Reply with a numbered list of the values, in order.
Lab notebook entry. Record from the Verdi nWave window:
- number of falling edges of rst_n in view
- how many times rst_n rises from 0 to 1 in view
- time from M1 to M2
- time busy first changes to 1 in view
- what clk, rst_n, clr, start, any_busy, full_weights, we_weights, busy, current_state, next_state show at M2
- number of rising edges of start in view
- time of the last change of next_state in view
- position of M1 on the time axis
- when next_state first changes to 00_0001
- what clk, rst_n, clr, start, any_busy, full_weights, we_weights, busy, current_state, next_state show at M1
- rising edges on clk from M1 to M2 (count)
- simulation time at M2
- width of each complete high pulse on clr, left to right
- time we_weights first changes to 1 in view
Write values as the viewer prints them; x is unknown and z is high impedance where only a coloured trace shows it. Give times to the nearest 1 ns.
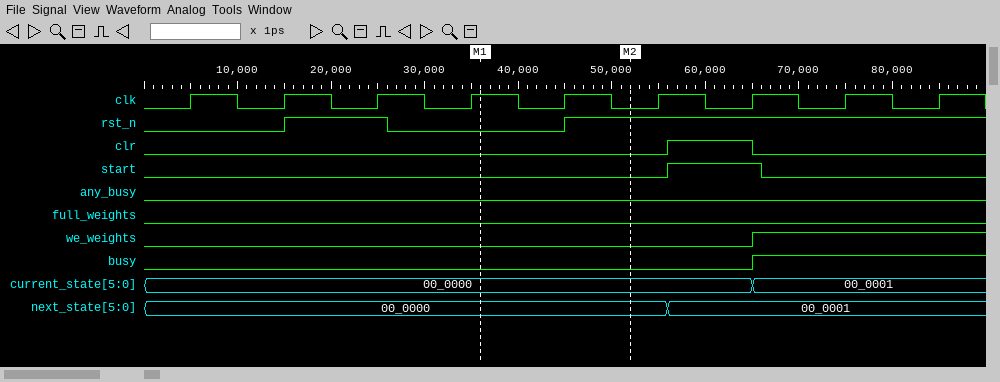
1. 1
2. 2
3. 16 ns
4. 65 ns
5. clk=0, rst_n=1, clr=0, start=0, any_busy=0, full_weights=0, we_weights=0, busy=0, current_state=00_0000, next_state=00_0000
6. 1
7. 56 ns
8. 36 ns
9. 56 ns
10. clk=1, rst_n=0, clr=0, start=0, any_busy=0, full_weights=0, we_weights=0, busy=0, current_state=00_0000, next_state=00_0000
11. 1
12. 52 ns
13. 9 ns
14. 65 ns
